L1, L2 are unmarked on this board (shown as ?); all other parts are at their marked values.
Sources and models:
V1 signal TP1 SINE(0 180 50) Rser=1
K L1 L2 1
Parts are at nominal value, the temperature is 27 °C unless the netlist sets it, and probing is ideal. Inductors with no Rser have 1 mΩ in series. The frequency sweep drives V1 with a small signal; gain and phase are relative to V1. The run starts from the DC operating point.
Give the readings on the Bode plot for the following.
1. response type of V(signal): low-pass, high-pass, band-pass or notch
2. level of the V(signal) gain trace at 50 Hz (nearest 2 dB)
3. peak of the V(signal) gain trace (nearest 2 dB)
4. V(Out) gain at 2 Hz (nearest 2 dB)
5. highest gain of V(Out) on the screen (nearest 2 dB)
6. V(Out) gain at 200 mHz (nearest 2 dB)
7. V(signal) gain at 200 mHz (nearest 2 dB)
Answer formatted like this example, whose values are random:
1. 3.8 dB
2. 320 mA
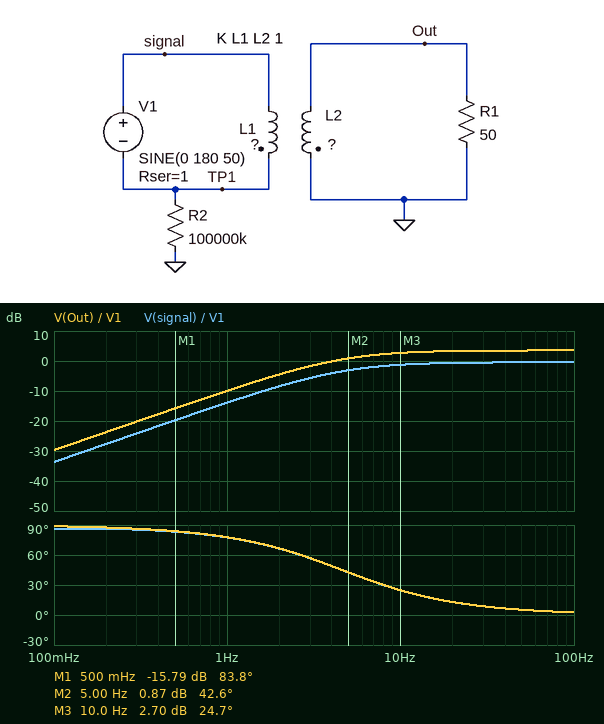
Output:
1. high-pass
2. 0 dB
3. 0 dB
4. -4 dB
5. 4 dB
6. -24 dB
7. -28 dB
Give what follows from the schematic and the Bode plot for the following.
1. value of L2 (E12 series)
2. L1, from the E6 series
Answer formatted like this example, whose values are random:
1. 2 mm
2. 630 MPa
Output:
1. 82 mH
2. 33 mH
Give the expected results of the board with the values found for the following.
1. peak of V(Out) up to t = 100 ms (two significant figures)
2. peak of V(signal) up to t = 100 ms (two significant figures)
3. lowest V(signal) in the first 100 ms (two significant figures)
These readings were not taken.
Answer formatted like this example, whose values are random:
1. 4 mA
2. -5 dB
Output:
1. 270 V
2. 170 V
3. -180 V
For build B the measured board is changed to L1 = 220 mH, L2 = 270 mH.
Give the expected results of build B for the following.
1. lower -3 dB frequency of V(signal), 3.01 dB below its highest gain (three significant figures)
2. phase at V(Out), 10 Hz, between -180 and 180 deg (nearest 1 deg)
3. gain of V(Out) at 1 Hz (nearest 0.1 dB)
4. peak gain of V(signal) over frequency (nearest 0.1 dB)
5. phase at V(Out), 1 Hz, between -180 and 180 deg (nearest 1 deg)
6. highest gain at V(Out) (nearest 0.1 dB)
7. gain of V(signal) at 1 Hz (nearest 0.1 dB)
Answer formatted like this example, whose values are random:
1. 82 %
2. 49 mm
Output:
1. 707 mHz
2. 4 deg
3. -1.1 dB
4. -0.2 dB
5. 35 deg
6. 0.7 dB
7. -2.0 dB
